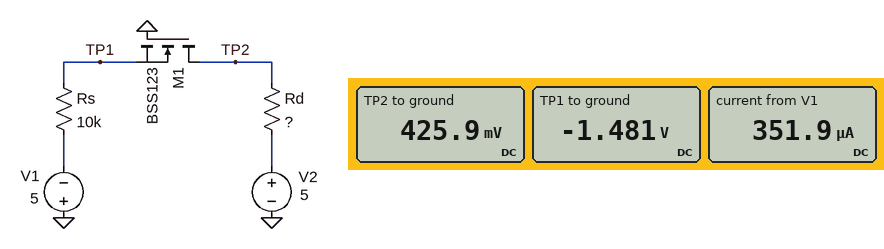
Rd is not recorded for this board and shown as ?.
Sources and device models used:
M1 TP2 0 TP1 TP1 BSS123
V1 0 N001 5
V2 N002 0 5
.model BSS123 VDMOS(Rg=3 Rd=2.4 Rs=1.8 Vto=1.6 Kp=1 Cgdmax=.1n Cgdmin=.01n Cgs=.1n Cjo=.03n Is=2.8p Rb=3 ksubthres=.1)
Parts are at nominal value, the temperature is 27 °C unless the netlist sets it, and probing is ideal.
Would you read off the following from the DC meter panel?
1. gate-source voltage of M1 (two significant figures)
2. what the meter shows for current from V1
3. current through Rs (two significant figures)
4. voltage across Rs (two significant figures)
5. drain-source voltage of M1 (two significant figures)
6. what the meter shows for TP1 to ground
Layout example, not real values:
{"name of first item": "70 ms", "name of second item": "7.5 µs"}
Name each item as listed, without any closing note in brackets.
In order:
{"gate-source voltage of M1": "1.5 V", "what the meter shows for current from V1": "351.9 µA", "current through Rs": "350 µA", "voltage across Rs": "3.5 V", "drain-source voltage of M1": "1.9 V", "what the meter shows for TP1 to ground": "-1.481 V"}
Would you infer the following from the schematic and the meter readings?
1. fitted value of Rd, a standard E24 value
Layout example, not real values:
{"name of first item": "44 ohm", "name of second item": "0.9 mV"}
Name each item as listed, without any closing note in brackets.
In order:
{"fitted value of Rd, a standard E24 value": "13 kΩ"}
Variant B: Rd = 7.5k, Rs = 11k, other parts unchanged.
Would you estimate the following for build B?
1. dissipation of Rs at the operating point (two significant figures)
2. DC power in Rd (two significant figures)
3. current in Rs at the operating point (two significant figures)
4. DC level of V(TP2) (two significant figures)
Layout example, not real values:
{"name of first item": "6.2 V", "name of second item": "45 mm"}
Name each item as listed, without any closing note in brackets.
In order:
{"dissipation of Rs at the operating point": "1.1 mW", "DC power in Rd": "770 µW", "current in Rs at the operating point": "320 µA", "DC level of V(TP2)": "2.6 V"}
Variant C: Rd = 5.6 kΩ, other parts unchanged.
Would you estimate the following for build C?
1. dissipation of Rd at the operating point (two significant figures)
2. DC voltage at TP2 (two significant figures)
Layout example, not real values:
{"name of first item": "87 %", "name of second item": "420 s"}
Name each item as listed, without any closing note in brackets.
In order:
{"dissipation of Rd at the operating point": "690 µW", "DC voltage at TP2": "3.0 V"}
